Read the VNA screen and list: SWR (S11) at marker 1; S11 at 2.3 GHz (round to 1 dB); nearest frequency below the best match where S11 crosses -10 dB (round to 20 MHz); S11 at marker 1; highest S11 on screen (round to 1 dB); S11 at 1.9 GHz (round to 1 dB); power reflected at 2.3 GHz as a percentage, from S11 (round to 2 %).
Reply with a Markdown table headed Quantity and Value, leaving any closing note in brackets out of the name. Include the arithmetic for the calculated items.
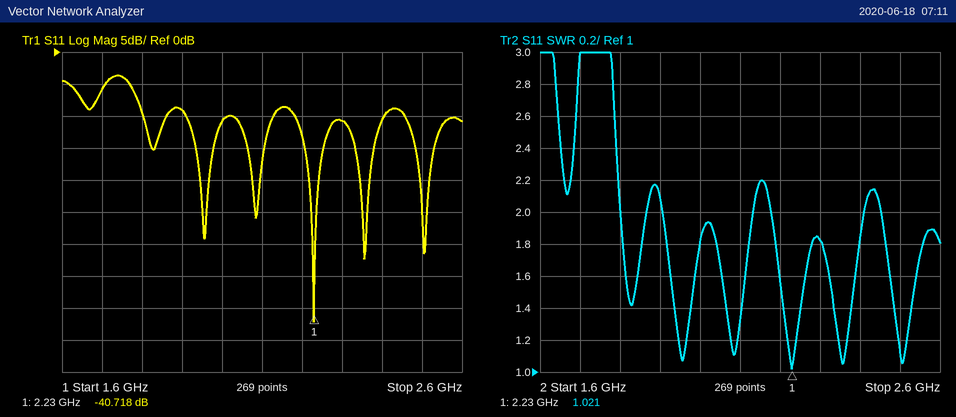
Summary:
| Quantity | Value |
|---|---|
| SWR (S11) at marker 1 | 1.021 |
| S11 at 2.3 GHz | -11 dB |
| nearest frequency below the best match where S11 crosses -10 dB | 2.18 GHz |
| S11 at marker 1 | -40.718 dB |
| highest S11 on screen | -4 dB |
| S11 at 1.9 GHz | -9 dB |
| power reflected at 2.3 GHz as a percentage, from S11 | 10^(-11/10) ≈ 8 % |
